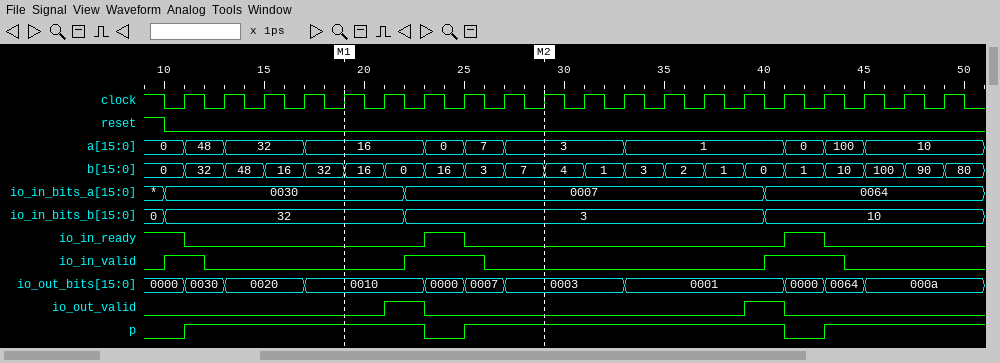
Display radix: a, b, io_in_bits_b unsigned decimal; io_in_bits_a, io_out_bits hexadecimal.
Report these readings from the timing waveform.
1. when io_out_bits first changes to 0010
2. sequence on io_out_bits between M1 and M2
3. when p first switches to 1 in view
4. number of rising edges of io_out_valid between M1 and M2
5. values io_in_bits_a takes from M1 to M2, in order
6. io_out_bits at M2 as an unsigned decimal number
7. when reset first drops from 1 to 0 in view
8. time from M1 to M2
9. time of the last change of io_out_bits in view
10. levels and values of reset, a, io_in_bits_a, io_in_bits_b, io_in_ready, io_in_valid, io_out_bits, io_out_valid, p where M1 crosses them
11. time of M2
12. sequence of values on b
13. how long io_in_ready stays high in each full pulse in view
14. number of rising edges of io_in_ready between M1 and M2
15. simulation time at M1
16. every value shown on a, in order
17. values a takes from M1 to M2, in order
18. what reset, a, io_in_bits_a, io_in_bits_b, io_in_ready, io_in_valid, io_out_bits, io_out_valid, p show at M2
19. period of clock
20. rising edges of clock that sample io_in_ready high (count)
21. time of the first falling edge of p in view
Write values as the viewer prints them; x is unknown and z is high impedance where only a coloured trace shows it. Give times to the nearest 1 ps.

17 ps
0010, 0000, 0007, 0003
11 ps
1
0030, 0007
3
10 ps
10 ps
45 ps
reset=0, a=16, io_in_bits_a=0030, io_in_bits_b=32, io_in_ready=0, io_in_valid=0, io_out_bits=0010, io_out_valid=0, p=1
29 ps
0, 32, 48, 16, 32, 16, 0, 16, 3, 7, 4, 1, 3, 2, 1, 0, 1, 10, 100, 90, 80
2 ps, 2 ps
1
19 ps
0, 48, 32, 16, 0, 7, 3, 1, 0, 100, 10
16, 0, 7, 3
reset=0, a=3, io_in_bits_a=0007, io_in_bits_b=3, io_in_ready=0, io_in_valid=0, io_out_bits=0003, io_out_valid=0, p=1
2 ps
3
23 ps
